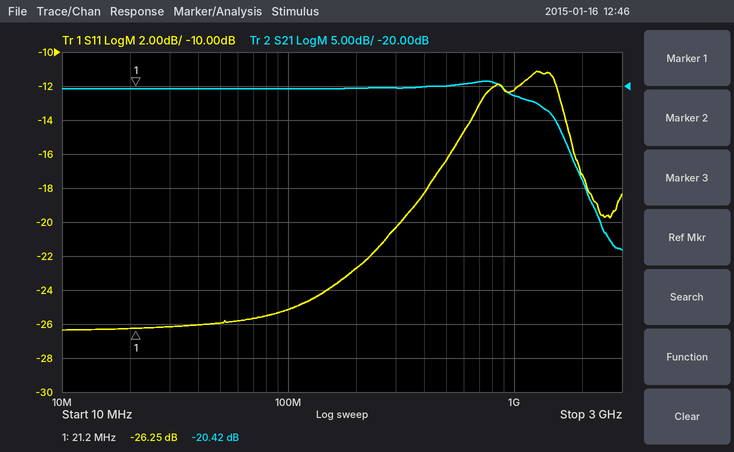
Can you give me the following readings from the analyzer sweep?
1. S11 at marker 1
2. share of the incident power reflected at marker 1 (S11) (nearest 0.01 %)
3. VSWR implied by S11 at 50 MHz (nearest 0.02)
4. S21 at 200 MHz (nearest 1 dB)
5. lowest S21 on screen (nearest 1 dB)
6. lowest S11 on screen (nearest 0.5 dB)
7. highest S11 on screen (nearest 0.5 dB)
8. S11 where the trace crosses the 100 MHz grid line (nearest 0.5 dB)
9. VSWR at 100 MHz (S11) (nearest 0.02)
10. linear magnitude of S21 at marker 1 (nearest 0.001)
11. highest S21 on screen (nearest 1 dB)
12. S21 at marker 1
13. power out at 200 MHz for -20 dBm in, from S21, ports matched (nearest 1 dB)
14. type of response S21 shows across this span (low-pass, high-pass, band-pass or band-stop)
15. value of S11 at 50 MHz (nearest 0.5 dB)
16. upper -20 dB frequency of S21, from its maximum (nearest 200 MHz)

-26.25 dB
0.24 %
1.10
-20 dB
-44 dB
-26.5 dB
-11.0 dB
-25.0 dB
1.12
0.095
-19 dB
-20.42 dB
-40 dBm
low-pass
-26.0 dB
2.4 GHz
